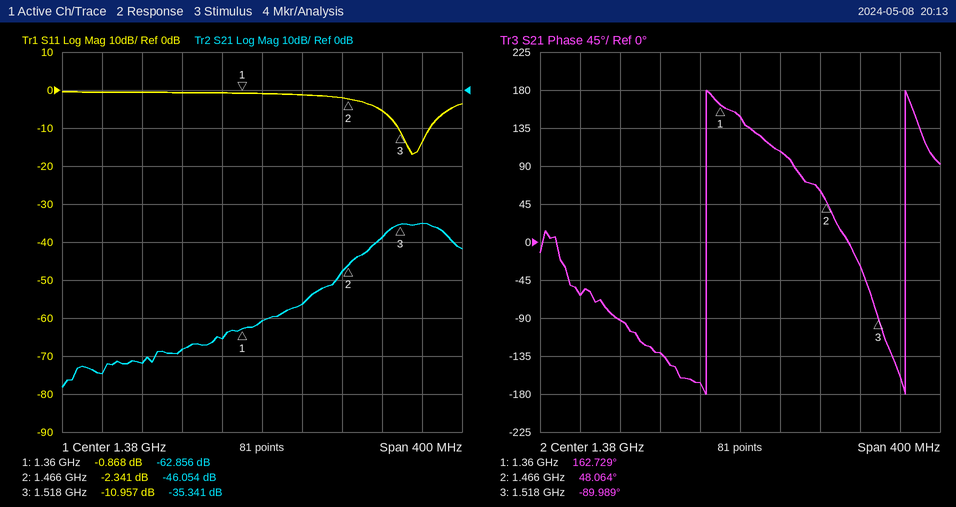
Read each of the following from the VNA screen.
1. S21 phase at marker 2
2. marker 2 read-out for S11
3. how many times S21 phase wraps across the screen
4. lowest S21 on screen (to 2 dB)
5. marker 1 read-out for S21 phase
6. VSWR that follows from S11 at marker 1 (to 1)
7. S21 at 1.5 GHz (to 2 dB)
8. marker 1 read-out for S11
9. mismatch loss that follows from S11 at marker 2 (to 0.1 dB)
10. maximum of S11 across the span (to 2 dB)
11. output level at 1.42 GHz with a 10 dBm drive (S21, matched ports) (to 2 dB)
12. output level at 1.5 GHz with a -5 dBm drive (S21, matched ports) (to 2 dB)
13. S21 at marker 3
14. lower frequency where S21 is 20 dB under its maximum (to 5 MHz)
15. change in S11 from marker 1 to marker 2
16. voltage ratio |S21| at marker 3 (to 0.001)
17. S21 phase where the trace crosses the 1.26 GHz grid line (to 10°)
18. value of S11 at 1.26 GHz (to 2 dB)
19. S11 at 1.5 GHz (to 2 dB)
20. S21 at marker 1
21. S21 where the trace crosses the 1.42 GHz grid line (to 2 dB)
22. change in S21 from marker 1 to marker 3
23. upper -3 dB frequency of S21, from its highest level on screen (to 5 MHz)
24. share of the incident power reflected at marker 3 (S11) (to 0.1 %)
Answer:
48.064°
-2.341 dB
2
-78 dB
162.729°
20
-38 dB
-0.868 dB
3.8 dB
0 dB
-46 dBm
-44 dBm
-35.341 dB
1.425 GHz
-1.473 dB
0.017
-90°
0 dB
-6 dB
-62.856 dB
-56 dB
27.515 dB
1.565 GHz
8.0 %
